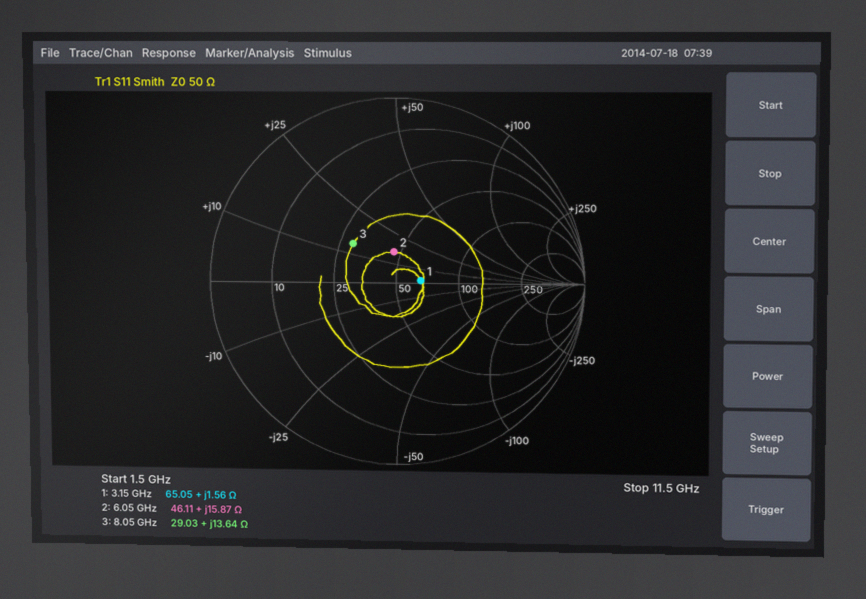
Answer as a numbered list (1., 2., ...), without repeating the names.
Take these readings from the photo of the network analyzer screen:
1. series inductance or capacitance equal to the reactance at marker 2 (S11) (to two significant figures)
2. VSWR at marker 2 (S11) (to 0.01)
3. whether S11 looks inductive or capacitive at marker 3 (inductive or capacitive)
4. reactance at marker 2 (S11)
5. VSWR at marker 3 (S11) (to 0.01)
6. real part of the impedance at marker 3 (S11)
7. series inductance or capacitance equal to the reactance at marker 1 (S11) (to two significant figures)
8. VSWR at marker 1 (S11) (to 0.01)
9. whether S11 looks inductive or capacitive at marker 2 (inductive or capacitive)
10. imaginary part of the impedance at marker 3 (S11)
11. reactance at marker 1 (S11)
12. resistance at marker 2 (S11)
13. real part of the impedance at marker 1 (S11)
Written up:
1. 420 pH
2. 1.40
3. inductive
4. +15.87 Ω
5. 1.91
6. 29.03 Ω
7. 79 pH
8. 1.30
9. inductive
10. +13.64 Ω
11. +1.56 Ω
12. 46.11 Ω
13. 65.05 Ω
